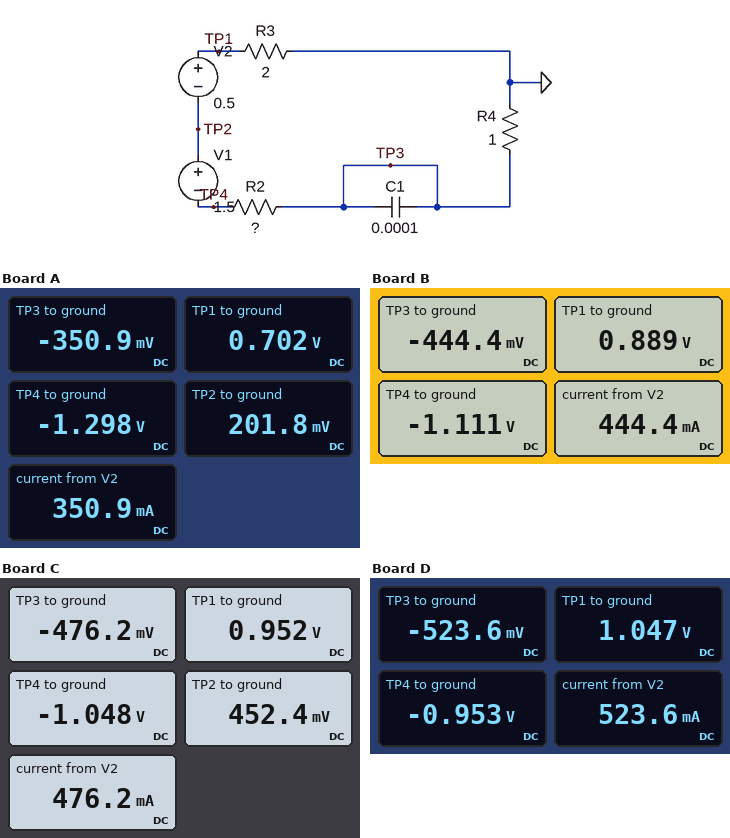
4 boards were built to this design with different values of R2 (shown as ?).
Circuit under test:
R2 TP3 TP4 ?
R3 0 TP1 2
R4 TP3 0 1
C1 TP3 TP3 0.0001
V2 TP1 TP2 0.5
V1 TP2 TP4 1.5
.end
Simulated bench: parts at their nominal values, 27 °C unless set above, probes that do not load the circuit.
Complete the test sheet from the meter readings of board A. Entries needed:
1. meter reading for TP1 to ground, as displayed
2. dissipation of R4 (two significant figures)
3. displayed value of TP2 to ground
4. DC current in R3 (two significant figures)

0.702 V
120 mW
201.8 mV
350 mA
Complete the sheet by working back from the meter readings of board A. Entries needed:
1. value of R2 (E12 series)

2.7 Ω
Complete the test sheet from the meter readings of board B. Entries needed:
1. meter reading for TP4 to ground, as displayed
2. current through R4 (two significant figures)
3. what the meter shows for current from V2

-1.111 V
440 mA
444.4 mA
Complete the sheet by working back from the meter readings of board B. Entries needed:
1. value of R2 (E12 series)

1.5 Ω
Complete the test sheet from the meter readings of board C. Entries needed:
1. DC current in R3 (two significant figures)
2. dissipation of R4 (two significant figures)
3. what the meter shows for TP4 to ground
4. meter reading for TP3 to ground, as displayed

480 mA
230 mW
-1.048 V
-476.2 mV
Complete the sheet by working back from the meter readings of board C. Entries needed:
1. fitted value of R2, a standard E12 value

1.2 Ω
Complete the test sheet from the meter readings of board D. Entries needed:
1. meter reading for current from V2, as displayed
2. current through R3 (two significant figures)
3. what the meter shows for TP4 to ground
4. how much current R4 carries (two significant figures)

523.6 mA
520 mA
-0.953 V
520 mA
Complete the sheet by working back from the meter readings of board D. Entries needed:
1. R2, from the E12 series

0.82 Ω
